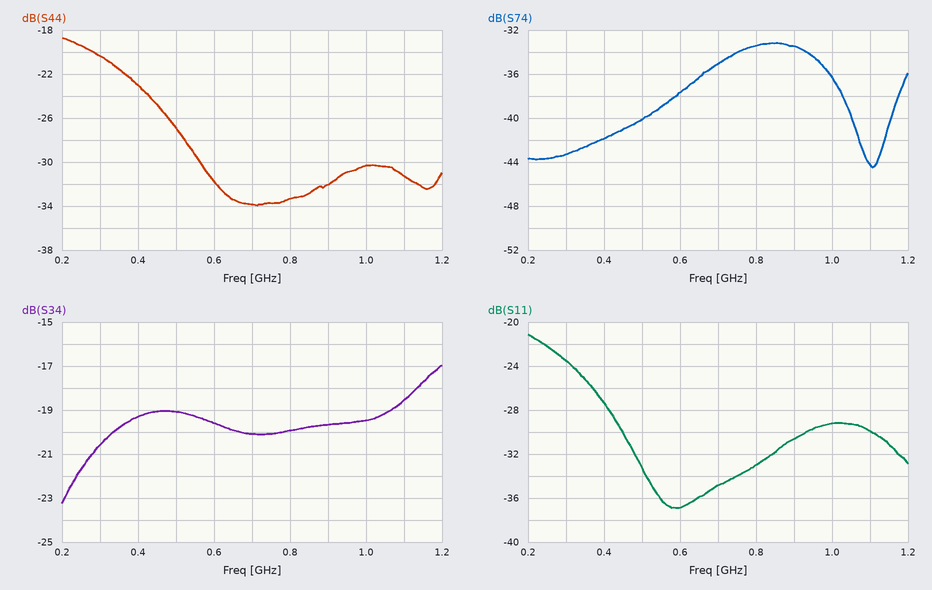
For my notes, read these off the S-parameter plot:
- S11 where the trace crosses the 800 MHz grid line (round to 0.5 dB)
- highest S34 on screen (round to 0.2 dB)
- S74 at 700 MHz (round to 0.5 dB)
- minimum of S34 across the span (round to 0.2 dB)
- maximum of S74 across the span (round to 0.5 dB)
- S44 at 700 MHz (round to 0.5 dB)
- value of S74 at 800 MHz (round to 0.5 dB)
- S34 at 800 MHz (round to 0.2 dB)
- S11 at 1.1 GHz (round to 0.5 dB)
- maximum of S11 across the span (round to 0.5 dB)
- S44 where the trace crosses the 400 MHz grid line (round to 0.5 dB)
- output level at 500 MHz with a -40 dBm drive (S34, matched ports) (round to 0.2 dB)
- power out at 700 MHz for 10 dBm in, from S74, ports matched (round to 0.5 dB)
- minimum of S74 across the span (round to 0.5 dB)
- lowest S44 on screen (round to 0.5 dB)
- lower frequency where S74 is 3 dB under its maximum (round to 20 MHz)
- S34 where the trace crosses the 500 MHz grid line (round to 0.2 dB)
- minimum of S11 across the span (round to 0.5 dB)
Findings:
-33.0 dB
-17.0 dB
-35.0 dB
-23.2 dB
-33.0 dB
-34.0 dB
-33.5 dB
-20.0 dB
-30.0 dB
-21.0 dB
-23.0 dB
-59.0 dBm
-25.0 dBm
-44.5 dB
-34.0 dB
660 MHz
-19.0 dB
-37.0 dB
